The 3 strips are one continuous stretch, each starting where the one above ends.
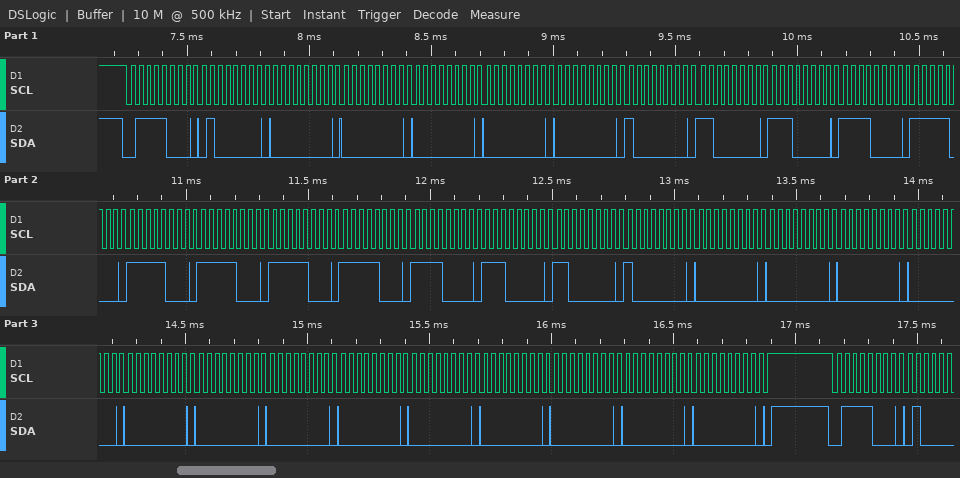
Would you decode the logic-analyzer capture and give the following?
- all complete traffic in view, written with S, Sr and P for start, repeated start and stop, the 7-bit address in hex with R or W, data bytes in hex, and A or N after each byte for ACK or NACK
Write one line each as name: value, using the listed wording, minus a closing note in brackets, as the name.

all complete traffic in view, written with S, Sr and P for start, repeated start and stop, the 7-bit address in hex with R or W, data bytes in hex, and A or N after each byte for ACK or NACK: S 3CW A 40 A 00 A 00 A 00 A 00 A 00 A 80 A C0 A E0 A F0 A F8 A F8 A F8 A F8 A F8 A F0 A E0 A C0 A 80 A 00 A 00 A 00 A 00 A 00 A 00 A 00 A 00 A 00 A 00 A 00 A 00 A 00 A P S 3CW A
